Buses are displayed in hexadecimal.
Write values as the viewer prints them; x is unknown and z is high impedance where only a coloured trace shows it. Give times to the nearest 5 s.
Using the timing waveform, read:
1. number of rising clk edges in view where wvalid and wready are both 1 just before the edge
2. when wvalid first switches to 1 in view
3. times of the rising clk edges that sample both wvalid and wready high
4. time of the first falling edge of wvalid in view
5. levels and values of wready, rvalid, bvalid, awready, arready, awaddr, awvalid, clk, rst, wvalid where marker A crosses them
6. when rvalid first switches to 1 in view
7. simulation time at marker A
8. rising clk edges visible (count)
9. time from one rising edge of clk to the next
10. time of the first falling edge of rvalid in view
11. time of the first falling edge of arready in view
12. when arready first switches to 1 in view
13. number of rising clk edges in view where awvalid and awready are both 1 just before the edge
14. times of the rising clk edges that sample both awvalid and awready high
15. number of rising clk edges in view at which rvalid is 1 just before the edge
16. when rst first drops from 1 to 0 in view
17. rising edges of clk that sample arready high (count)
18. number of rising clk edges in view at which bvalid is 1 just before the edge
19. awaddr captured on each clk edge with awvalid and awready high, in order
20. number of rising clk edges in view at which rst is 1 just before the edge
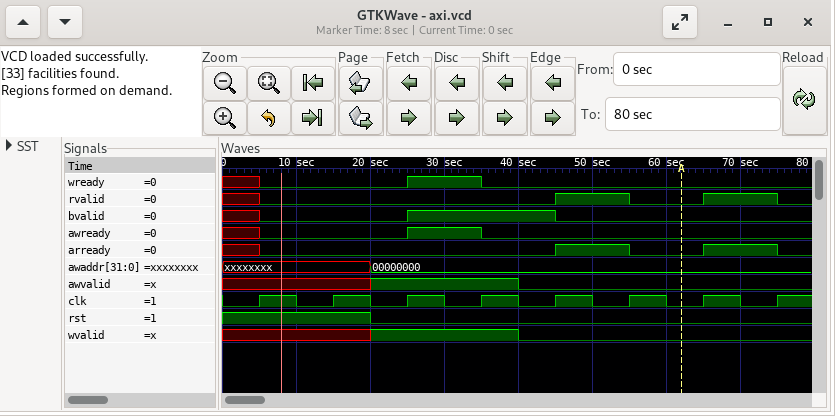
1
20 s
35 s
40 s
wready=0, rvalid=0, bvalid=0, awready=0, arready=0, awaddr=00000000, awvalid=0, clk=0, rst=0, wvalid=0
45 s
60 s
8
10 s
55 s
55 s
45 s
1
35 s
2
20 s
2
2
00000000
2
